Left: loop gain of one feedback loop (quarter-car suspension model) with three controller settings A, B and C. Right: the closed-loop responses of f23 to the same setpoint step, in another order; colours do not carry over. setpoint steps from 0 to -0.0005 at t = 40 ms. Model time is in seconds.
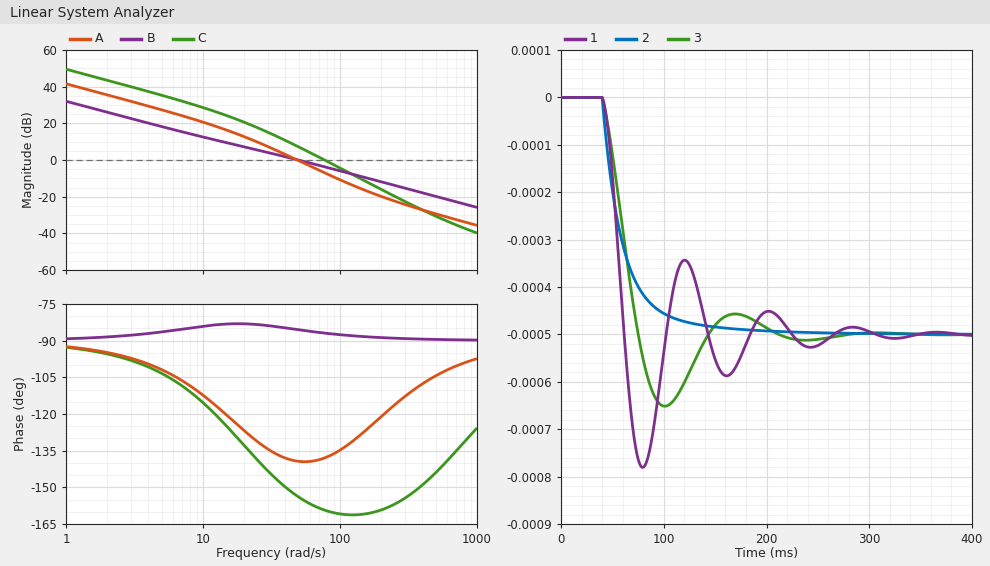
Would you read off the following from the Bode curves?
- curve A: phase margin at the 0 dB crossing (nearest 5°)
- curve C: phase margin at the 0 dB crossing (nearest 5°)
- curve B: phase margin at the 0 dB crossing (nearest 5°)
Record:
40°
20°
95°
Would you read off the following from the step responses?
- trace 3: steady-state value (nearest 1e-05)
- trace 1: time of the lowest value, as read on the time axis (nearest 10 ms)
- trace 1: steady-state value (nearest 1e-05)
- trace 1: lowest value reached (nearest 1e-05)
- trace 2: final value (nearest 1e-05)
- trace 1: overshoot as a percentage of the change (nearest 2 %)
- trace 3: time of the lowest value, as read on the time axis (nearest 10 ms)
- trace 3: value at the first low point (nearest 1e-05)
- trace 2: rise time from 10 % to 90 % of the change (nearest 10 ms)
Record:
-0.00050
80 ms
-0.00050
-0.00078
-0.00050
56 %
100 ms
-0.00065
50 ms
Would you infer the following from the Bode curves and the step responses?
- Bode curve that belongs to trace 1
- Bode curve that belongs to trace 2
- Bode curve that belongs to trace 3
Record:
C
B
A
